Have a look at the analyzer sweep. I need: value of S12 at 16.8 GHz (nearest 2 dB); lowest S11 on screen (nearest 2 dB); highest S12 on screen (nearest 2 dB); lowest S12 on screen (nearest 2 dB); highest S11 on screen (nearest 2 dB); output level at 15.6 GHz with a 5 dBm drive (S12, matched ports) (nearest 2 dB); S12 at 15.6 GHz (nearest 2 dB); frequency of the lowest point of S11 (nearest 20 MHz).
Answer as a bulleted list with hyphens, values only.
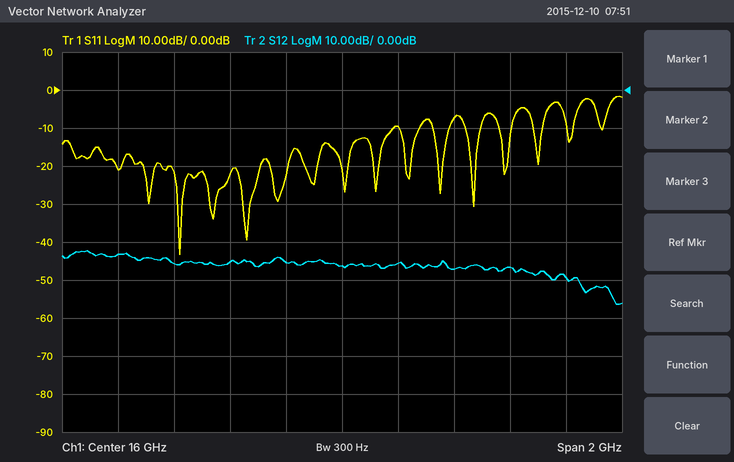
- -50 dB
- -44 dB
- -42 dB
- -56 dB
- -2 dB
- -40 dBm
- -46 dB
- 15.42 GHz
